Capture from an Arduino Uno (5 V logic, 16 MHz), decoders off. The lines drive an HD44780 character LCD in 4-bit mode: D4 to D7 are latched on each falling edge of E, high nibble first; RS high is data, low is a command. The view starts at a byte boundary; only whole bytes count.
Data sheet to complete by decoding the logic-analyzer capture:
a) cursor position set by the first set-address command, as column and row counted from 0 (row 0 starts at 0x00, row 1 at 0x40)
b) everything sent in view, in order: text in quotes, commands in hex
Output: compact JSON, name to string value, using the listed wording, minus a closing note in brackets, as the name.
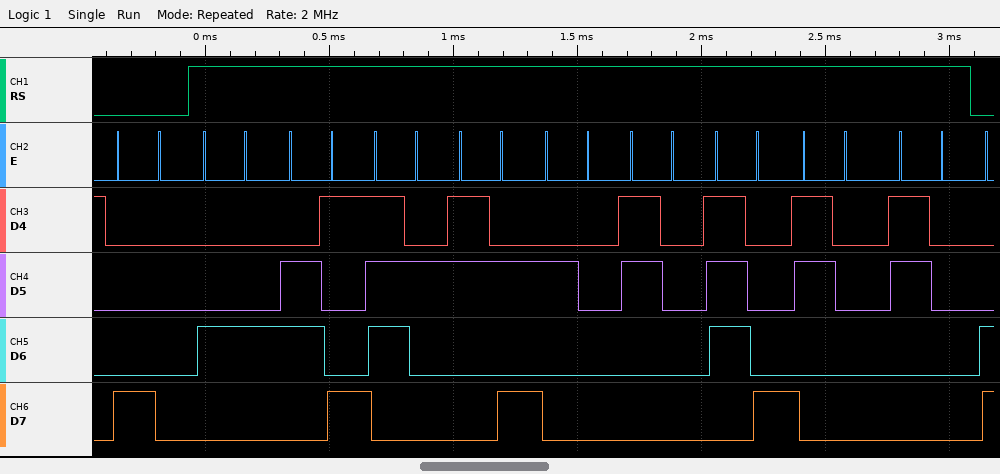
{"cursor position set by the first set-address command, as column and row counted from 0": "column 0, row 0", "everything sent in view, in order: text in quotes, commands in hex": "0x80 \"Dir: 0x00\""}
